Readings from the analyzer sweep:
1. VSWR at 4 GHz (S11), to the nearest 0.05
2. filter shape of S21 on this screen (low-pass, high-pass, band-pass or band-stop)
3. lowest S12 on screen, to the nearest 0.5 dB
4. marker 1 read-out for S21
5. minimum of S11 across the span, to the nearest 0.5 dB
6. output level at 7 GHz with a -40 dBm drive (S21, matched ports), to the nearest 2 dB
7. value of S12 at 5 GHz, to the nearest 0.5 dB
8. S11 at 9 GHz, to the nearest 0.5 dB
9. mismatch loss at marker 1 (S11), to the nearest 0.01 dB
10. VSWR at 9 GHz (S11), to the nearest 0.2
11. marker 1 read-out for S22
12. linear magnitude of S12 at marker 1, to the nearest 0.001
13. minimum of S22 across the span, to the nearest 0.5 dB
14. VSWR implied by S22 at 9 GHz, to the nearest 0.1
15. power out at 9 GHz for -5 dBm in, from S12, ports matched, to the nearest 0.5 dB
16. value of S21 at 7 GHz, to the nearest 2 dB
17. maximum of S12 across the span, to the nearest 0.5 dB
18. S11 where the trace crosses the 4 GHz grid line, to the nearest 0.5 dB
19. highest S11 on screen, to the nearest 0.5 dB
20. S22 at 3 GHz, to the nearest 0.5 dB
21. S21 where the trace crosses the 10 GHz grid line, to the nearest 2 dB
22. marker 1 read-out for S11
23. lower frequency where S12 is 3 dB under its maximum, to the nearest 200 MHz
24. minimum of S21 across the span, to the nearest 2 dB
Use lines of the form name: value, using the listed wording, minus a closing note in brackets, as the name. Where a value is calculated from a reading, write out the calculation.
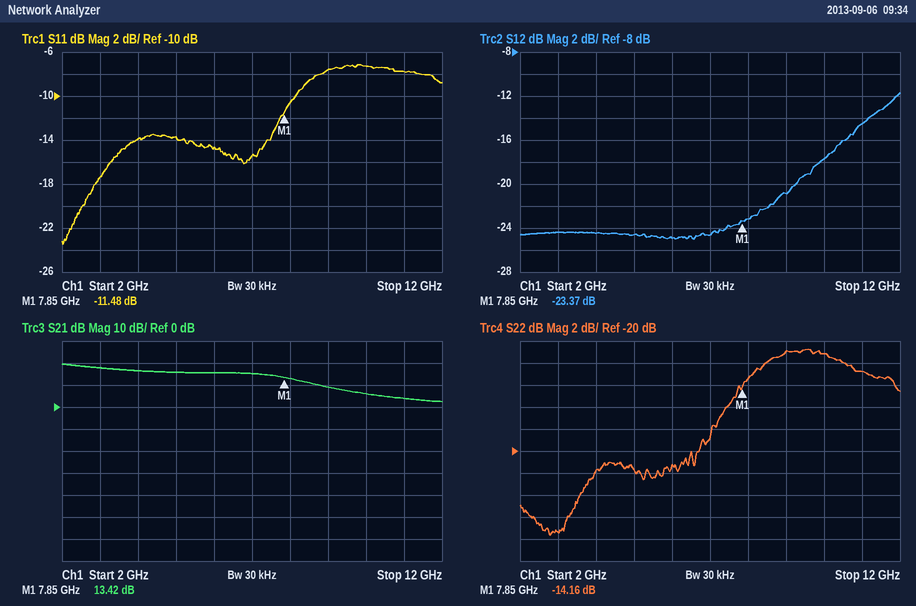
VSWR at 4 GHz (S11), to the nearest 0.05: |Γ| = 10^(-14/20) = 0.1995; VSWR = (1 + 0.1995)/(1 − 0.1995) ≈ 1.50
filter shape of S21 on this screen: low-pass
lowest S12 on screen, to the nearest 0.5 dB: -25.0 dB
marker 1 read-out for S21: 13.42 dB
minimum of S11 across the span, to the nearest 0.5 dB: -23.5 dB
output level at 7 GHz with a -40 dBm drive (S21, matched ports), to the nearest 2 dB: -40 dBm + (16 dB) = -24 dBm
value of S12 at 5 GHz, to the nearest 0.5 dB: -24.5 dB
S11 at 9 GHz, to the nearest 0.5 dB: -7.5 dB
mismatch loss at marker 1 (S11), to the nearest 0.01 dB: −10 log10(1 − 10^(-11.48/10)) ≈ 0.32 dB
VSWR at 9 GHz (S11), to the nearest 0.2: |Γ| = 10^(-7.5/20) = 0.4217; VSWR = (1 + 0.4217)/(1 − 0.4217) ≈ 2.46, so 2.4 to the nearest 0.2
marker 1 read-out for S22: -14.16 dB
linear magnitude of S12 at marker 1, to the nearest 0.001: 10^(-23.37/20) ≈ 0.068
minimum of S22 across the span, to the nearest 0.5 dB: -27.5 dB
VSWR implied by S22 at 9 GHz, to the nearest 0.1: |Γ| = 10^(-11/20) = 0.2818; VSWR = (1 + 0.2818)/(1 − 0.2818) ≈ 1.8
power out at 9 GHz for -5 dBm in, from S12, ports matched, to the nearest 0.5 dB: -5 dBm + (-21.0 dB) = -26.0 dBm
value of S21 at 7 GHz, to the nearest 2 dB: 16 dB
maximum of S12 across the span, to the nearest 0.5 dB: -11.5 dB
S11 where the trace crosses the 4 GHz grid line, to the nearest 0.5 dB: -14.0 dB
highest S11 on screen, to the nearest 0.5 dB: -7.0 dB
S22 at 3 GHz, to the nearest 0.5 dB: -27.5 dB
S21 where the trace crosses the 10 GHz grid line, to the nearest 2 dB: 6 dB
marker 1 read-out for S11: -11.48 dB
lower frequency where S12 is 3 dB under its maximum, to the nearest 200 MHz: 11.0 GHz
minimum of S21 across the span, to the nearest 2 dB: 2 dB
